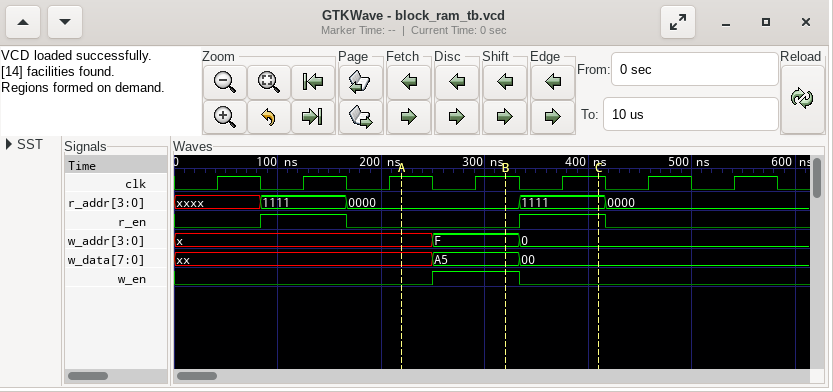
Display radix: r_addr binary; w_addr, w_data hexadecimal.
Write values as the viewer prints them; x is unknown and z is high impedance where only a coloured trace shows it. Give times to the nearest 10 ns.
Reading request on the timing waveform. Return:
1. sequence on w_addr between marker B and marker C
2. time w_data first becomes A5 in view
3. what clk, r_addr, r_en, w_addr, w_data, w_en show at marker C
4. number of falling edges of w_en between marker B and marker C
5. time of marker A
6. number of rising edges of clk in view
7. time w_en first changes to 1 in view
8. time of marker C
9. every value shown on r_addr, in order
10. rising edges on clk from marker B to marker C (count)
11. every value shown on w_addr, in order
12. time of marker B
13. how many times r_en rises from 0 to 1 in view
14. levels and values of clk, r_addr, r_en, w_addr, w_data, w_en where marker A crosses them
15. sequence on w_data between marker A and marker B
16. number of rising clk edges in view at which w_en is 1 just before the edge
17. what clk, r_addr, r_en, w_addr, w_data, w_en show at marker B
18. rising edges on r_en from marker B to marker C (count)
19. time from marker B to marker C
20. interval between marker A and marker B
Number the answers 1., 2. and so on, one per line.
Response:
1. F, 0
2. 250 ns
3. clk=1, r_addr=1111, r_en=1, w_addr=0, w_data=00, w_en=0
4. 1
5. 220 ns
6. 7
7. 250 ns
8. 410 ns
9. xxxx, 1111, 0000, 1111, 0000
10. 1
11. x, F, 0
12. 320 ns
13. 2
14. clk=1, r_addr=0000, r_en=0, w_addr=x, w_data=xx, w_en=0
15. xx, A5
16. 1
17. clk=1, r_addr=0000, r_en=0, w_addr=F, w_data=A5, w_en=1
18. 1
19. 90 ns
20. 100 ns
